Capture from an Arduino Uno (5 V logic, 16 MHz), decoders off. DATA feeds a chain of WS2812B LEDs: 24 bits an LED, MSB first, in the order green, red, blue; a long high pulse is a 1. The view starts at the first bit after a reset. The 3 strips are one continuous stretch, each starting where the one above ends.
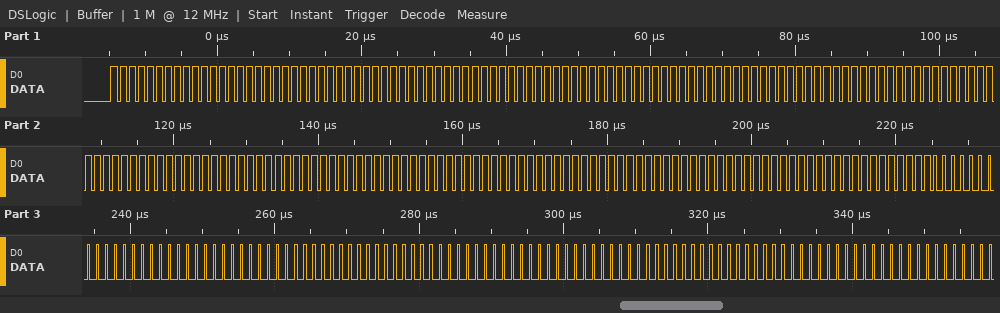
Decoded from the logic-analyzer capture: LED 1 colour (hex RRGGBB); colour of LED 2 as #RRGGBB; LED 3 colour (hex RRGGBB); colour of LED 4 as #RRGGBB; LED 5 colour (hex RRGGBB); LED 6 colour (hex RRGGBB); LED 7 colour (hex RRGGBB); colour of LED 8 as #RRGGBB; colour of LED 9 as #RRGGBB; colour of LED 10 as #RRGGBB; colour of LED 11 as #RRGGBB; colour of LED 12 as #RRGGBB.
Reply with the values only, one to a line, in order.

#FFFFFF
#FFFFFF
#FFFFFF
#FFFFFF
#FFFFFF
#FFFFFF
#FFFFFF
#FFFFFF
#000000
#000000
#000000
#000000
